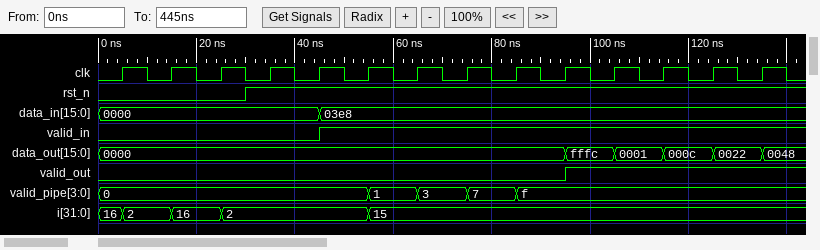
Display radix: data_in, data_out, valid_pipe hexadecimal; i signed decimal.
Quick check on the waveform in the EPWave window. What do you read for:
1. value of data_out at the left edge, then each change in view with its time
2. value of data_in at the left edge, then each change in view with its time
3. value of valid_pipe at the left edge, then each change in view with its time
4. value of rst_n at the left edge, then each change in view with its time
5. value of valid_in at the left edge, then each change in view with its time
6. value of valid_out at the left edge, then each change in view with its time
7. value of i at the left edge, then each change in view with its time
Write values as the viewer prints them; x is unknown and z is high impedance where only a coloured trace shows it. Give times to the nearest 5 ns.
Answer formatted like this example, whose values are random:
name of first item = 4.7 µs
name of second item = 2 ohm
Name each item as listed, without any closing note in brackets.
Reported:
value of data_out at the left edge, then each change in view with its time = 0000, fffc at 95 ns, 0001 at 105 ns, 000c at 115 ns, 0022 at 125 ns, 0048 at 135 ns
value of data_in at the left edge, then each change in view with its time = 0000, 03e8 at 45 ns
value of valid_pipe at the left edge, then each change in view with its time = 0, 1 at 55 ns, 3 at 65 ns, 7 at 75 ns, f at 85 ns
value of rst_n at the left edge, then each change in view with its time = 0, 1 at 30 ns
value of valid_in at the left edge, then each change in view with its time = 0, 1 at 45 ns
value of valid_out at the left edge, then each change in view with its time = 0, 1 at 95 ns
value of i at the left edge, then each change in view with its time = 16, 2 at 5 ns, 16 at 15 ns, 2 at 25 ns, 15 at 55 ns
